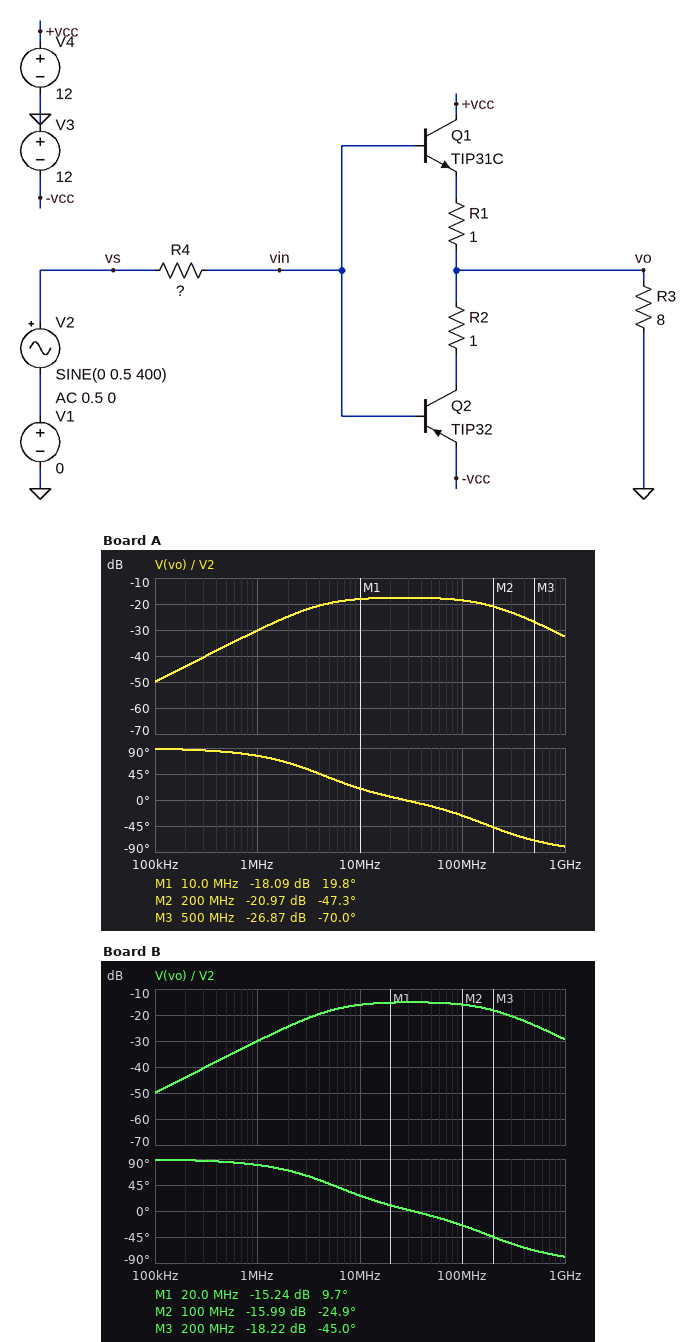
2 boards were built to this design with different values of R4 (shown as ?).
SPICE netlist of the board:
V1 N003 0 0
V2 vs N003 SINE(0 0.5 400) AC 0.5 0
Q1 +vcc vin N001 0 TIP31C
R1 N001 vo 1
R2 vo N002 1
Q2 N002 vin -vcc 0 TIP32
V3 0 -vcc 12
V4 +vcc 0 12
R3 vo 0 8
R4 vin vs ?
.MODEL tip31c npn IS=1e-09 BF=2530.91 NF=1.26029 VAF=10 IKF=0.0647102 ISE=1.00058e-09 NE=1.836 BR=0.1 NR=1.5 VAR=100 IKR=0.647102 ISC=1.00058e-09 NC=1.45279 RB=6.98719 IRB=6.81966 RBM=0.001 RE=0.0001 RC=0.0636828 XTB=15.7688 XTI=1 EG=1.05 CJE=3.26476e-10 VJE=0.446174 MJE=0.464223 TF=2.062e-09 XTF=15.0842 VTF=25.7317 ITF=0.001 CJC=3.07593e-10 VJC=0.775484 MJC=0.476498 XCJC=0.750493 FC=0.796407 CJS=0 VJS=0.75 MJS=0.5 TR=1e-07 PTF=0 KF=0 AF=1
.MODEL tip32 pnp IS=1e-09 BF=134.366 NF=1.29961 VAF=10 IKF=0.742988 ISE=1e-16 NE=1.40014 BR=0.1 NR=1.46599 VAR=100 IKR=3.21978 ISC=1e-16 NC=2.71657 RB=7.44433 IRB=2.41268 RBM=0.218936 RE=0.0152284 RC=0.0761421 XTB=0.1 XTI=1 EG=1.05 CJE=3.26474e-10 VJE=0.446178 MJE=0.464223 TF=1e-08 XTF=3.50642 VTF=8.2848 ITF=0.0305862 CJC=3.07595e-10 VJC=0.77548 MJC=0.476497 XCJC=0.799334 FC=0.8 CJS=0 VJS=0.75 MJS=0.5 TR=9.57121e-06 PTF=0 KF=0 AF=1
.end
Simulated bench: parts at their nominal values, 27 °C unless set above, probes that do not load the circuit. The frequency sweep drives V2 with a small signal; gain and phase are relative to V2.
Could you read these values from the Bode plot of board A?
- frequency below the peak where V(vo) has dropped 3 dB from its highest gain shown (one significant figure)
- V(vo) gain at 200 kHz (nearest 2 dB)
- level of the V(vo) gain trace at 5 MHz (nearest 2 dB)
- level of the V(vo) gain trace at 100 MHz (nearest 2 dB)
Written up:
4 MHz
-44 dB
-20 dB
-18 dB
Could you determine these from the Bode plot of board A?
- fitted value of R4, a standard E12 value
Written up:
39 Ω
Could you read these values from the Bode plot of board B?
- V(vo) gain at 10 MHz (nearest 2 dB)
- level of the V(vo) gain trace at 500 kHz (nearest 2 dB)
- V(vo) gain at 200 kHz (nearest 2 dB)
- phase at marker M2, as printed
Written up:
-16 dB
-36 dB
-44 dB
-24.9 deg
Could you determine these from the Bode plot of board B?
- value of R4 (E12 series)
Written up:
27 Ω
